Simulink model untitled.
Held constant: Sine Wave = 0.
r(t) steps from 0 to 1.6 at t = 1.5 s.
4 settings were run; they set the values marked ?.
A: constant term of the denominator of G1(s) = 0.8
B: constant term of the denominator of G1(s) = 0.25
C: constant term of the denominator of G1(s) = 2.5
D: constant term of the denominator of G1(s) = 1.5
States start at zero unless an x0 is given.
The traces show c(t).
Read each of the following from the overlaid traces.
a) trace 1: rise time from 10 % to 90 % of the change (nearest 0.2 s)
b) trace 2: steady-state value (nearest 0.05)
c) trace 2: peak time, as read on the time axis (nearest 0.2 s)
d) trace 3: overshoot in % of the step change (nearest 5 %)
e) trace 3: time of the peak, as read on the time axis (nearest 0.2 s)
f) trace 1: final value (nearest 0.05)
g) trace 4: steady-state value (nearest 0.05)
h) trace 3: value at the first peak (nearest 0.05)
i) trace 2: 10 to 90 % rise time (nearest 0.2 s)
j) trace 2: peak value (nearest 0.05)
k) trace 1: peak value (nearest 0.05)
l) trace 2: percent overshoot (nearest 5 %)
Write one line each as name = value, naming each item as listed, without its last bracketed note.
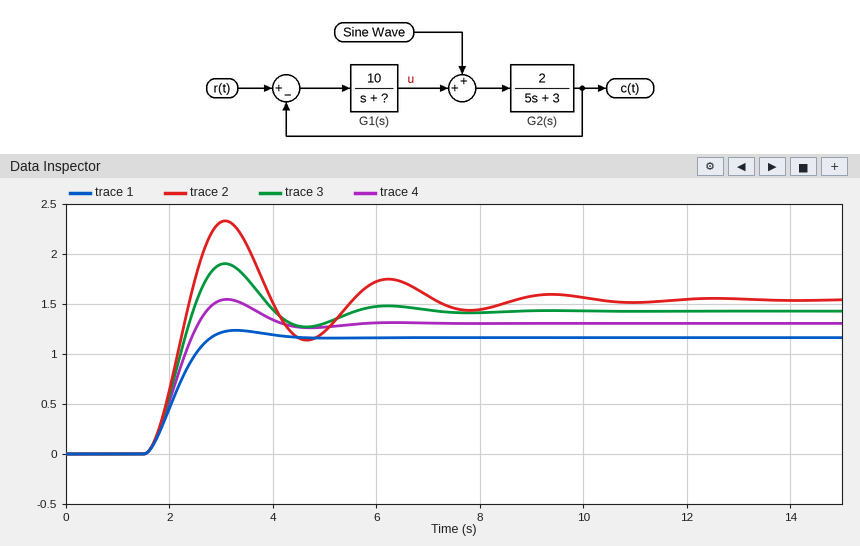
trace 1: rise time from 10 % to 90 % of the change = 0.8 s
trace 2: steady-state value = 1.55
trace 2: peak time, as read on the time axis = 3.0 s
trace 3: overshoot in % of the step change = 35 %
trace 3: time of the peak, as read on the time axis = 3.0 s
trace 1: final value = 1.15
trace 4: steady-state value = 1.30
trace 3: value at the first peak = 1.90
trace 2: 10 to 90 % rise time = 0.6 s
trace 2: peak value = 2.35
trace 1: peak value = 1.25
trace 2: percent overshoot = 50 %
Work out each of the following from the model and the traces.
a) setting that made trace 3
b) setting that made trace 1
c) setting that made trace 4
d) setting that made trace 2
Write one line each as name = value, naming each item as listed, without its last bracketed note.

setting that made trace 3 = A
setting that made trace 1 = C
setting that made trace 4 = D
setting that made trace 2 = B
